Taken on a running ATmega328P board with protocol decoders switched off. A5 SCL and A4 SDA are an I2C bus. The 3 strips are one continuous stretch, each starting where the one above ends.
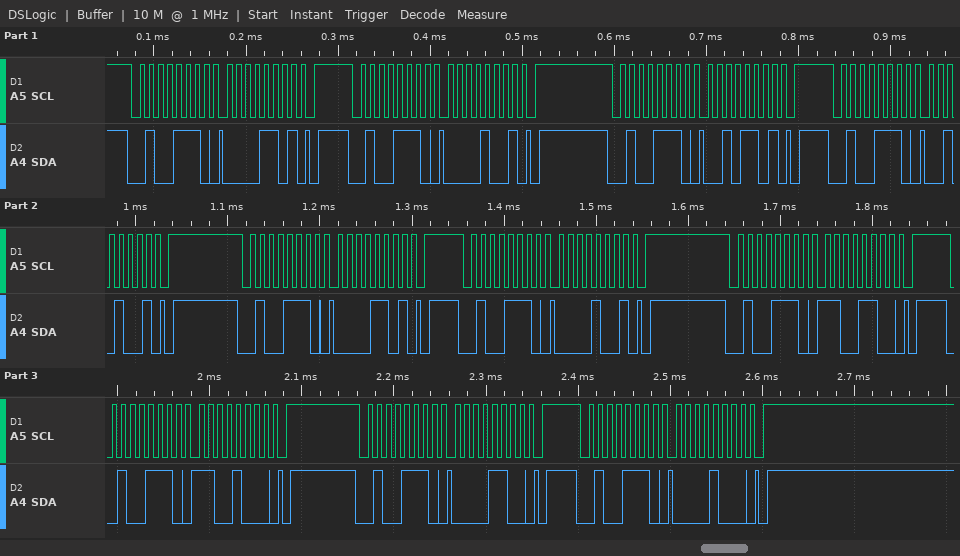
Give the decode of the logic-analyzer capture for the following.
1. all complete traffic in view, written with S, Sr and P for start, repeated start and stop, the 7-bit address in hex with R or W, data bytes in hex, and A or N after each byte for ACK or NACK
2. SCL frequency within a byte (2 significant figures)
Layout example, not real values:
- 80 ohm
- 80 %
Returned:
- S 27W A 0D A P S 27W A 09 A P S 27W A 2D A P S 27W A 29 A P S 27W A 0D A P S 27W A 09 A P S 27W A CC A P S 27W A C8 A P S 27W A 0C A P S 27W A 08 A P
- 100 kHz
